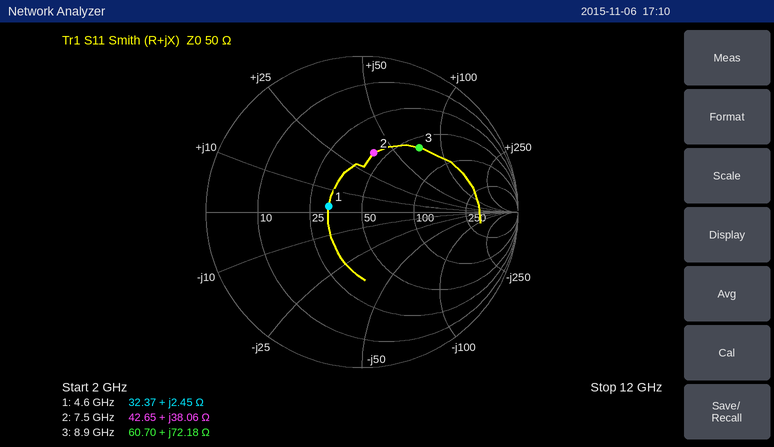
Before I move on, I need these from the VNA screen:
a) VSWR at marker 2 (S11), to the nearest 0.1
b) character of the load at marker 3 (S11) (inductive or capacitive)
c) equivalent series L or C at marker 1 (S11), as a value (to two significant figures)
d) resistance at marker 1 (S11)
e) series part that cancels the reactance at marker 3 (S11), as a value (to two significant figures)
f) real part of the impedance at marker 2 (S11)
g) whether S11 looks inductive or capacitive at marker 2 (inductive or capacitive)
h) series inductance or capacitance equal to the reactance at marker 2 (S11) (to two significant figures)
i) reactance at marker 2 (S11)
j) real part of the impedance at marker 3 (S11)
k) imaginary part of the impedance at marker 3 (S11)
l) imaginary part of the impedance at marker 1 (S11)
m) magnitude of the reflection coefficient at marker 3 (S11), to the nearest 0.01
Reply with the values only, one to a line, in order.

2.3
inductive
85 pH
32.37 Ω
250 fF
42.65 Ω
inductive
810 pH
+38.06 Ω
60.70 Ω
+72.18 Ω
+2.45 Ω
0.55
